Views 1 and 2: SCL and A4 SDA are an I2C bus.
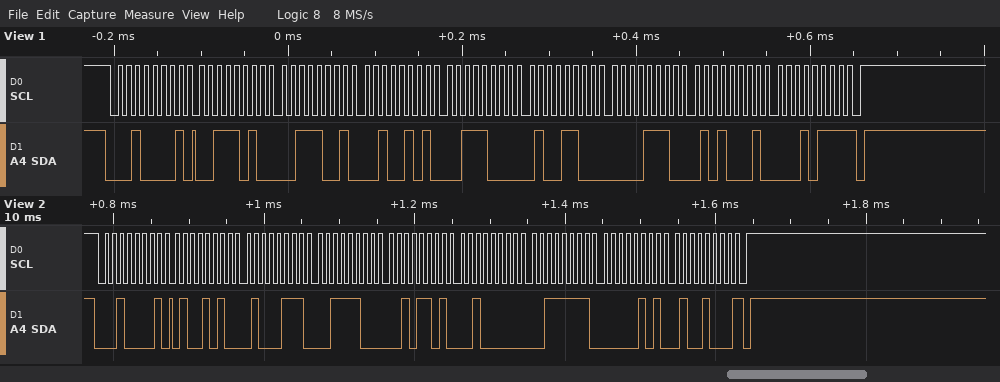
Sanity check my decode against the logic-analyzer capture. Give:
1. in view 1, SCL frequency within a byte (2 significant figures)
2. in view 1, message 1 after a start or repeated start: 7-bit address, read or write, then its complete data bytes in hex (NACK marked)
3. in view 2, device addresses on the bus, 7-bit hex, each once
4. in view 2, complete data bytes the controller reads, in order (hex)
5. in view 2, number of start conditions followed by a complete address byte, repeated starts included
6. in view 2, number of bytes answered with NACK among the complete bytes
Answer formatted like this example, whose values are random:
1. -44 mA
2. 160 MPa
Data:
1. 100 kHz
2. 0x10 read: 3A 39 25 38 4C 0E 51 17 NACK
3. 0x10
4. 4A 47 3C 2D 20 3F 05 48
5. 1
6. 1
